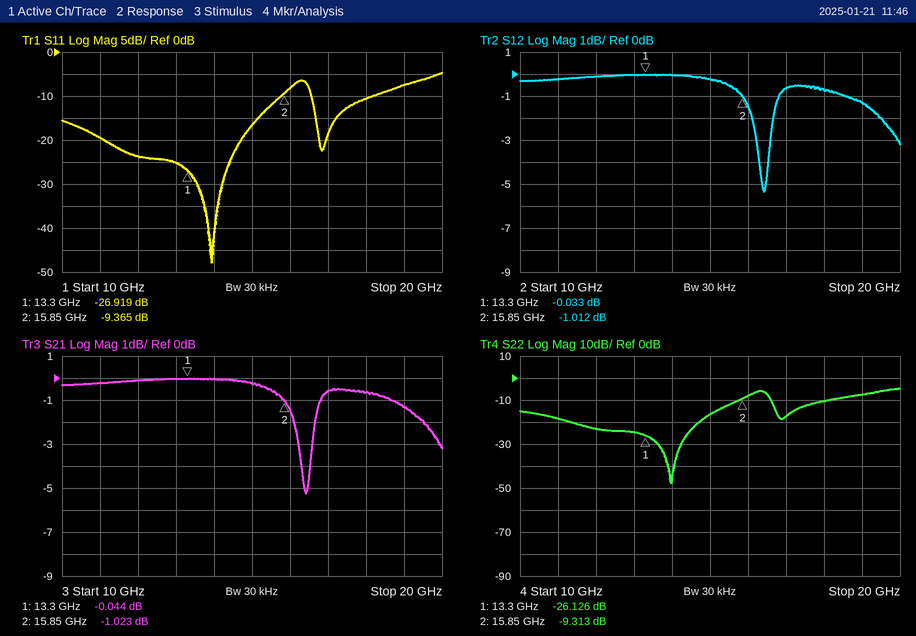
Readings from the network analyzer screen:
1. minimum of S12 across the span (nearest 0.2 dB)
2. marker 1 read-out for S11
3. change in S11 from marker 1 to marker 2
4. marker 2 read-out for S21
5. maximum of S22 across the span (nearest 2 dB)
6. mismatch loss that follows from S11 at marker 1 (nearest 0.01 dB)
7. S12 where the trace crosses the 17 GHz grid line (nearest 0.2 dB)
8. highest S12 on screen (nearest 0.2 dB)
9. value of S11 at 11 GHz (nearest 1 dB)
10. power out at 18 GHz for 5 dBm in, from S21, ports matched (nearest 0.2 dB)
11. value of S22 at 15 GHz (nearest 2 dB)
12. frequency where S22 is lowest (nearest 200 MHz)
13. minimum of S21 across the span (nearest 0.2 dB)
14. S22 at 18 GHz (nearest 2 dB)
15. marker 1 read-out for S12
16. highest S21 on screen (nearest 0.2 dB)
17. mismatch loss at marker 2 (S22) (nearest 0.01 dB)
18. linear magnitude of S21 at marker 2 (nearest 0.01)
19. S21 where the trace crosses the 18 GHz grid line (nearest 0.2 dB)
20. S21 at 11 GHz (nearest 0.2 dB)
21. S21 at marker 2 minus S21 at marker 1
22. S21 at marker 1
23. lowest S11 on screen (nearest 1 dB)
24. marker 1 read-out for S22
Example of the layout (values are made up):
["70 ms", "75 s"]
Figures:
["-5.4 dB", "-26.919 dB", "17.554 dB", "-1.023 dB", "-4 dB", "0.01 dB", "-0.6 dB", "0.0 dB", "-19 dB", "4.4 dBm", "-16 dB", "14.0 GHz", "-5.2 dB", "-10 dB", "-0.033 dB", "0.0 dB", "0.54 dB", "0.89", "-0.6 dB", "-0.2 dB", "-0.979 dB", "-0.044 dB", "-48 dB", "-26.126 dB"]
